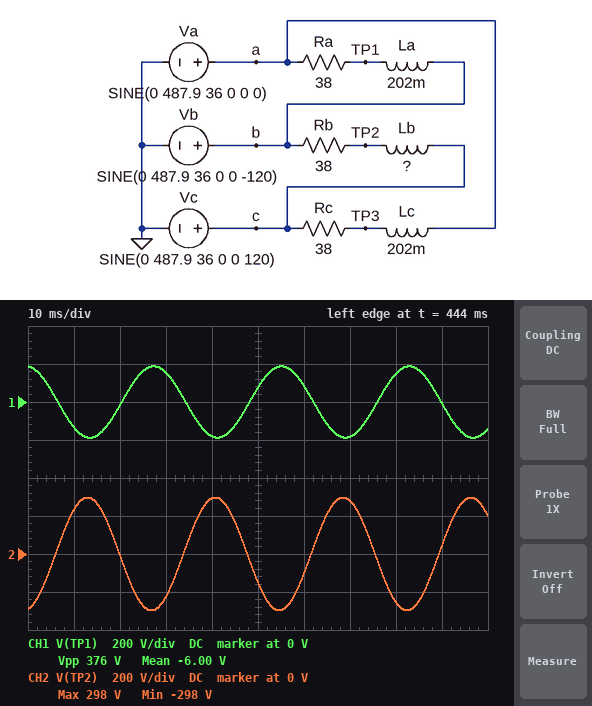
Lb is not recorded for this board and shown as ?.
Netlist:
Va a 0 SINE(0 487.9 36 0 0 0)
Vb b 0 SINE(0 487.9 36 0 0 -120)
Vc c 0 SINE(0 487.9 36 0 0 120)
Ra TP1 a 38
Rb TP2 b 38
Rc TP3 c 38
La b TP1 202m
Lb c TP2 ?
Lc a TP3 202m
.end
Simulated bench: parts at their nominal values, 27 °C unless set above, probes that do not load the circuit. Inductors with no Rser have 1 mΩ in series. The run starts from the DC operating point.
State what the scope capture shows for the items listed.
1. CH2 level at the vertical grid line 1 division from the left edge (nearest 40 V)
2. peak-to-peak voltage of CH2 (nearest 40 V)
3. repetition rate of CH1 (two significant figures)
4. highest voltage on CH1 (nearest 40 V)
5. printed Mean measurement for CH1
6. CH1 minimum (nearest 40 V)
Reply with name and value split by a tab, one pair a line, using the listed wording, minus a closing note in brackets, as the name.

CH2 level at the vertical grid line 1 division from the left edge	240 V
peak-to-peak voltage of CH2	600 V
repetition rate of CH1	36 Hz
highest voltage on CH1	200 V
printed Mean measurement for CH1	-6.00 V
CH1 minimum	-200 V
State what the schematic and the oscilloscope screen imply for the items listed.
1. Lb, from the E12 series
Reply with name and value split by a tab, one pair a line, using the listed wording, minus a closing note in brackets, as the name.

Lb, from the E12 series	390 mH
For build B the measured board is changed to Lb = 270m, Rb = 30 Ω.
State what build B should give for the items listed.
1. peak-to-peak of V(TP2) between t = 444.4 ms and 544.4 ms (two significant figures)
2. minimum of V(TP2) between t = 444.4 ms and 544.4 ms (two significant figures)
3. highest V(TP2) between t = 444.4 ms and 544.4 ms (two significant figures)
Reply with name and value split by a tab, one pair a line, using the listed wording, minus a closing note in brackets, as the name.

peak-to-peak of V(TP2) between t = 444.4 ms and 544.4 ms	550 V
minimum of V(TP2) between t = 444.4 ms and 544.4 ms	-270 V
highest V(TP2) between t = 444.4 ms and 544.4 ms	270 V
